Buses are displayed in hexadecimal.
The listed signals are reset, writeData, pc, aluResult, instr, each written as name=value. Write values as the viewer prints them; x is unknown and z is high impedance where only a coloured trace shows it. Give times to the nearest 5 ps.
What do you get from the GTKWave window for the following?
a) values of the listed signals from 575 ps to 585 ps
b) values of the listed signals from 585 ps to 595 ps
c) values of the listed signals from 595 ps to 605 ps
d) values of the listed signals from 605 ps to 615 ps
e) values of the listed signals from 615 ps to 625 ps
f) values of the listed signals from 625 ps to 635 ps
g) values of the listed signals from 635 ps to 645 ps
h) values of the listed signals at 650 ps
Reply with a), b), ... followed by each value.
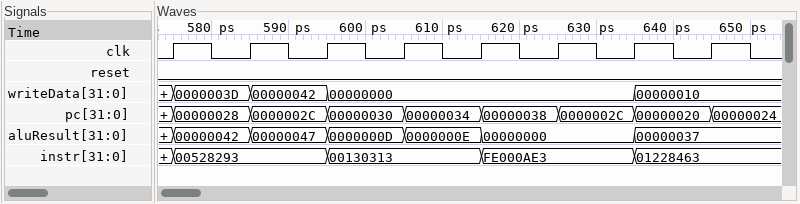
a) reset=0, writeData=0000003D, pc=00000028, aluResult=00000042, instr=00528293
b) reset=0, writeData=00000042, pc=0000002C, aluResult=00000047, instr=00528293
c) reset=0, writeData=00000000, pc=00000030, aluResult=0000000D, instr=00130313
d) reset=0, writeData=00000000, pc=00000034, aluResult=0000000E, instr=00130313
e) reset=0, writeData=00000000, pc=00000038, aluResult=00000000, instr=FE000AE3
f) reset=0, writeData=00000000, pc=0000002C, aluResult=00000000, instr=FE000AE3
g) reset=0, writeData=00000010, pc=00000020, aluResult=00000037, instr=01228463
h) reset=0, writeData=00000010, pc=00000024, aluResult=00000037, instr=01228463
